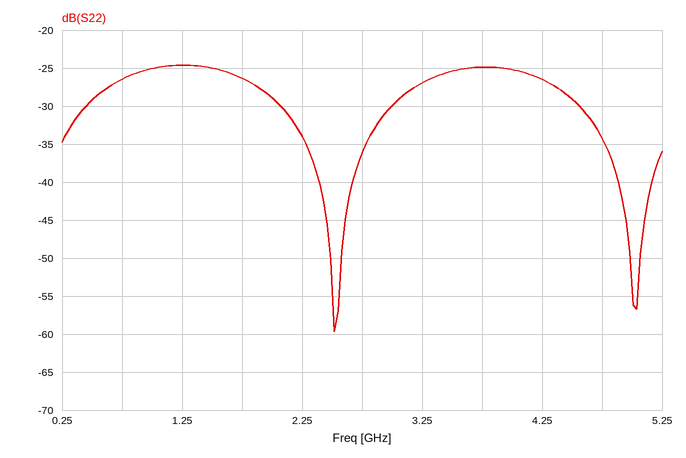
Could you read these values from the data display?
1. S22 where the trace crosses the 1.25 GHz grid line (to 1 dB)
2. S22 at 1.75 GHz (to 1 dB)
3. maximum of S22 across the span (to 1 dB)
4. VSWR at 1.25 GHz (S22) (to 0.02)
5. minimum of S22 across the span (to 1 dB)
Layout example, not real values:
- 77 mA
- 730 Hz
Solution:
- -25 dB
- -26 dB
- -25 dB
- 1.12
- -60 dB
